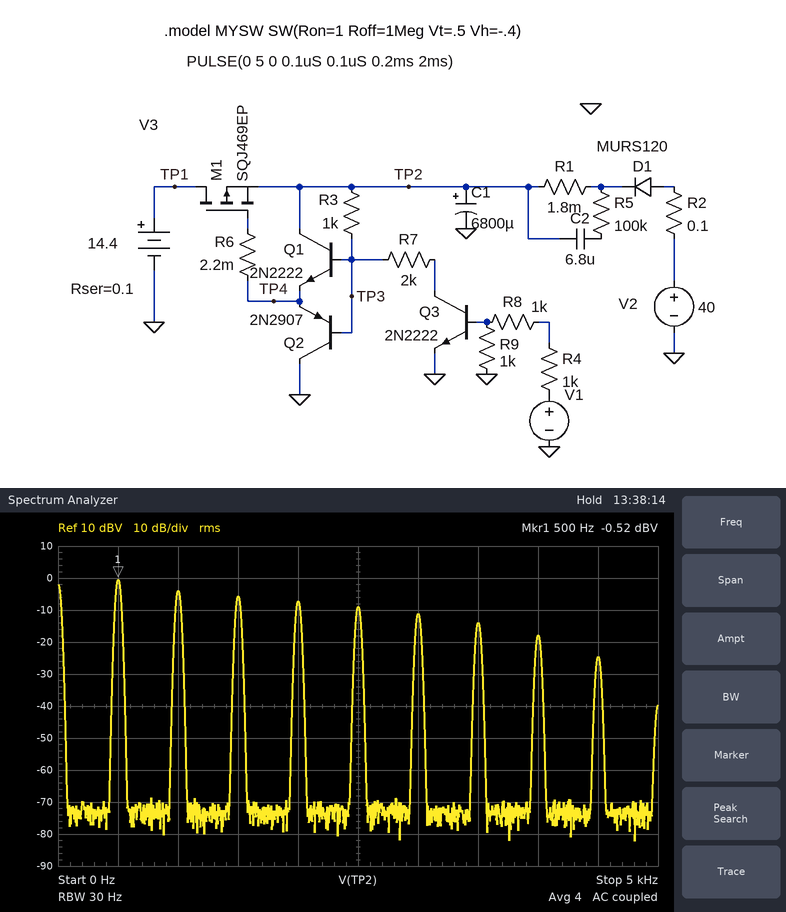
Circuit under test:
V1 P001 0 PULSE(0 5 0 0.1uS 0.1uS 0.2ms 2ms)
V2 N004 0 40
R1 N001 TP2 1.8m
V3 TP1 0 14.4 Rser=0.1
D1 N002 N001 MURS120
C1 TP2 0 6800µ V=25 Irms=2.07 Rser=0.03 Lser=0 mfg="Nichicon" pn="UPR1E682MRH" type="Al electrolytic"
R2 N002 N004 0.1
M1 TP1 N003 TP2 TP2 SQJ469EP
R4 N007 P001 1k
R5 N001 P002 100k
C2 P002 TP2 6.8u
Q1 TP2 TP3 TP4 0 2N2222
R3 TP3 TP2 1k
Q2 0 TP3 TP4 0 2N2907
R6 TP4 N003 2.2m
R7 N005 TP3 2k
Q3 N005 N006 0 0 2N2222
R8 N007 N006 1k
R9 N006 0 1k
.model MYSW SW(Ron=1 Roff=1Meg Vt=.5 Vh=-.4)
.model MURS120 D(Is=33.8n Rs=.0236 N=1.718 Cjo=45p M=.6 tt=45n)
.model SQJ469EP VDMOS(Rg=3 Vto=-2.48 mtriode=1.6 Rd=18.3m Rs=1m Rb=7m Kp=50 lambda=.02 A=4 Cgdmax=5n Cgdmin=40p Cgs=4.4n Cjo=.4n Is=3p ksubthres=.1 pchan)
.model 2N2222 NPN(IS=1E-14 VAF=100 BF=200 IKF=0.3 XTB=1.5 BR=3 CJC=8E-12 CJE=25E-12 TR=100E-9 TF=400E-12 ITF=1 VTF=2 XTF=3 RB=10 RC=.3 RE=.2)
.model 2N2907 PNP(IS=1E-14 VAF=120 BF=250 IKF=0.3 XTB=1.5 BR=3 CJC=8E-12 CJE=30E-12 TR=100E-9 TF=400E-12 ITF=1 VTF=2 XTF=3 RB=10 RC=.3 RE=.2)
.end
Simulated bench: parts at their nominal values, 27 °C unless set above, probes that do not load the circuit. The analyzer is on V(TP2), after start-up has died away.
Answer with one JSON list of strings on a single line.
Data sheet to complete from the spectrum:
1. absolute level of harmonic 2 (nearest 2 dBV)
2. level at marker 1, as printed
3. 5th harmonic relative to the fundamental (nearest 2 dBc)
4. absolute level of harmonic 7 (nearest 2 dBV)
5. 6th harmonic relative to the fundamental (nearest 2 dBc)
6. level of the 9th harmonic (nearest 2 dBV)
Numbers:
["-4 dBV", "-0.52 dBV", "-8 dBc", "-14 dBV", "-10 dBc", "-24 dBV"]
